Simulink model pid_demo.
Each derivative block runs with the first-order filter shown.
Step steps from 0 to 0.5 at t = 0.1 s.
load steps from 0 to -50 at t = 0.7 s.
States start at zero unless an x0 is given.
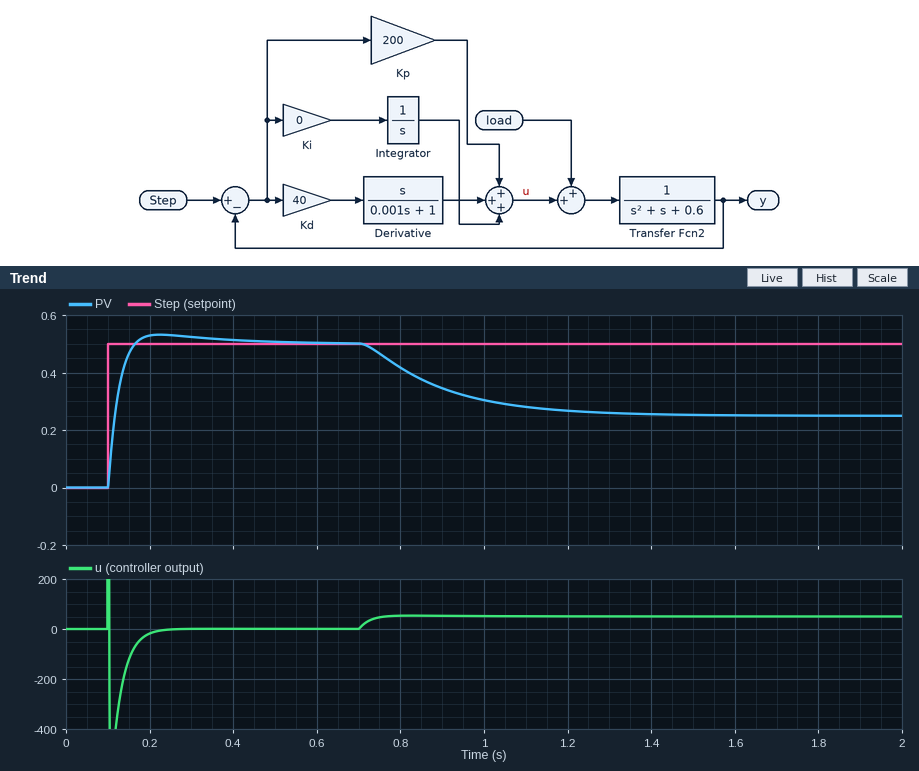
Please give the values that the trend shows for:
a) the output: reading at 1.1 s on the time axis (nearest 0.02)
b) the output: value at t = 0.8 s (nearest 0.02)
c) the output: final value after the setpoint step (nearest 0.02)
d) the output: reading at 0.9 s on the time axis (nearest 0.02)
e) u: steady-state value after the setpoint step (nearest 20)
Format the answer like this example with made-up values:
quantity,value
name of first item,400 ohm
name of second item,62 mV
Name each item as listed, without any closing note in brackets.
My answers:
quantity,value
the output: reading at 1.1 s on the time axis,0.28
the output: value at t = 0.8 s,0.42
the output: final value after the setpoint step,0.50
the output: reading at 0.9 s on the time axis,0.34
u: steady-state value after the setpoint step,0
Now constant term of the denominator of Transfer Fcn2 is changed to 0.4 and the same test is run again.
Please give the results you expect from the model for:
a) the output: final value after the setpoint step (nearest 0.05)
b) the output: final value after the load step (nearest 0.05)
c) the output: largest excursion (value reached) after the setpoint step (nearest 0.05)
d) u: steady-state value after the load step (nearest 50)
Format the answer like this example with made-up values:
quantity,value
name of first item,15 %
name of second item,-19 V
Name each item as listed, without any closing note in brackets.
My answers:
quantity,value
the output: final value after the setpoint step,0.50
the output: final value after the load step,0.25
the output: largest excursion (value reached) after the setpoint step,0.55
u: steady-state value after the load step,50
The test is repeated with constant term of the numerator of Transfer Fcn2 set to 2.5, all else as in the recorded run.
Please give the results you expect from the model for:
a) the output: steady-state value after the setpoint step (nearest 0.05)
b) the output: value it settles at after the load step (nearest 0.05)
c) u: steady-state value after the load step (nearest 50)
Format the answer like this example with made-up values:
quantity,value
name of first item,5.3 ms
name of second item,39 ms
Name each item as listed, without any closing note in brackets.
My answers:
quantity,value
the output: steady-state value after the setpoint step,0.50
the output: value it settles at after the load step,0.25
u: steady-state value after the load step,50
